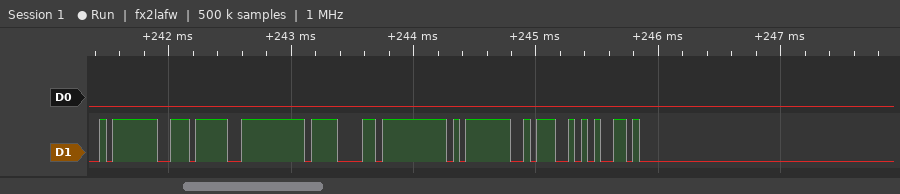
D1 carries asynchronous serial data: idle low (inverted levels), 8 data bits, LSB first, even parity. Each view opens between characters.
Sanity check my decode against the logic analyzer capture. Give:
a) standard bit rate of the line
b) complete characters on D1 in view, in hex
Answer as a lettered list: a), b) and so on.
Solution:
a) 19200 baud
b) 01, 04, 00, 78, 00, 01, B1, D3
